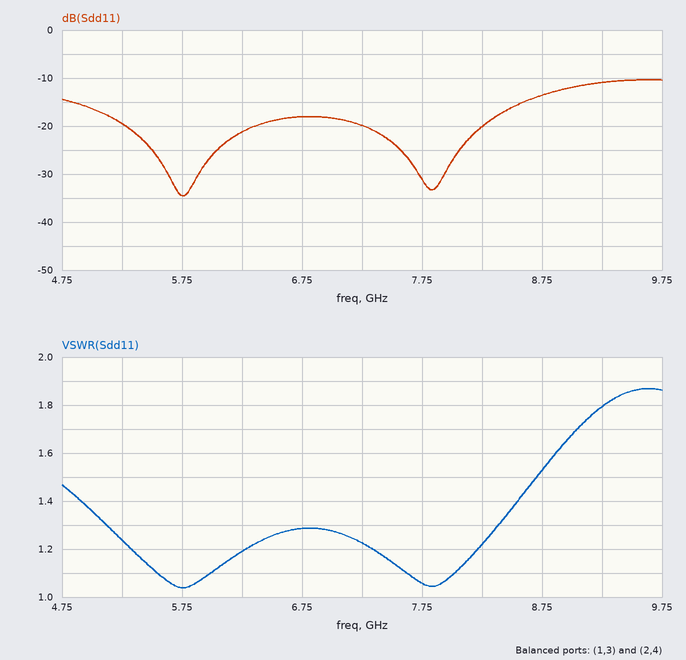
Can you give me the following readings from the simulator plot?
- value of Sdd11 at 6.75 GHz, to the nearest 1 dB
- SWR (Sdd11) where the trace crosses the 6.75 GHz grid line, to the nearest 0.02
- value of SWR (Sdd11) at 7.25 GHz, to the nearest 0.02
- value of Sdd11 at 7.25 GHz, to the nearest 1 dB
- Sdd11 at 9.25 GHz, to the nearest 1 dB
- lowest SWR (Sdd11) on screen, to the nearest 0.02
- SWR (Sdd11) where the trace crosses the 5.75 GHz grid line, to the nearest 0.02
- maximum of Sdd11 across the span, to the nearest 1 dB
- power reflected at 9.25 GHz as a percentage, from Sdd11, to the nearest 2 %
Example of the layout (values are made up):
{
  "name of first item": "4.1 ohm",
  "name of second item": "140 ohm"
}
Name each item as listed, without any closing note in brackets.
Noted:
{
  "value of Sdd11 at 6.75 GHz, to the nearest 1 dB": "-18 dB",
  "SWR (Sdd11) where the trace crosses the 6.75 GHz grid line, to the nearest 0.02": "1.28",
  "value of SWR (Sdd11) at 7.25 GHz, to the nearest 0.02": "1.22",
  "value of Sdd11 at 7.25 GHz, to the nearest 1 dB": "-20 dB",
  "Sdd11 at 9.25 GHz, to the nearest 1 dB": "-11 dB",
  "lowest SWR (Sdd11) on screen, to the nearest 0.02": "1.04",
  "SWR (Sdd11) where the trace crosses the 5.75 GHz grid line, to the nearest 0.02": "1.04",
  "maximum of Sdd11 across the span, to the nearest 1 dB": "-10 dB",
  "power reflected at 9.25 GHz as a percentage, from Sdd11, to the nearest 2 %": "8 %"
}
